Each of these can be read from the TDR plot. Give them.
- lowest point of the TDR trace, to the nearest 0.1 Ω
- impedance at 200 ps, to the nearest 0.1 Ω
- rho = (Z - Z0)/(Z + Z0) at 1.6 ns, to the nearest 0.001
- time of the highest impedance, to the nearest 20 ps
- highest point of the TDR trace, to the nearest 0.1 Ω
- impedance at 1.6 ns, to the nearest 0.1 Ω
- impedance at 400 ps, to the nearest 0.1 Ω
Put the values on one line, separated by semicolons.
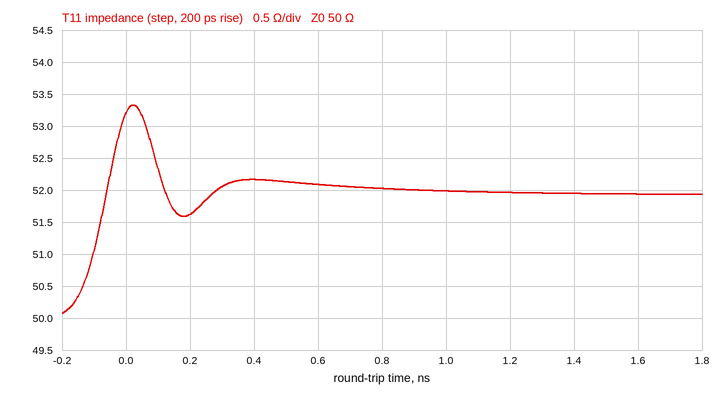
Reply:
50.1 Ω; 51.6 Ω; +0.019; 20 ps; 53.3 Ω; 51.9 Ω; 52.2 Ω
